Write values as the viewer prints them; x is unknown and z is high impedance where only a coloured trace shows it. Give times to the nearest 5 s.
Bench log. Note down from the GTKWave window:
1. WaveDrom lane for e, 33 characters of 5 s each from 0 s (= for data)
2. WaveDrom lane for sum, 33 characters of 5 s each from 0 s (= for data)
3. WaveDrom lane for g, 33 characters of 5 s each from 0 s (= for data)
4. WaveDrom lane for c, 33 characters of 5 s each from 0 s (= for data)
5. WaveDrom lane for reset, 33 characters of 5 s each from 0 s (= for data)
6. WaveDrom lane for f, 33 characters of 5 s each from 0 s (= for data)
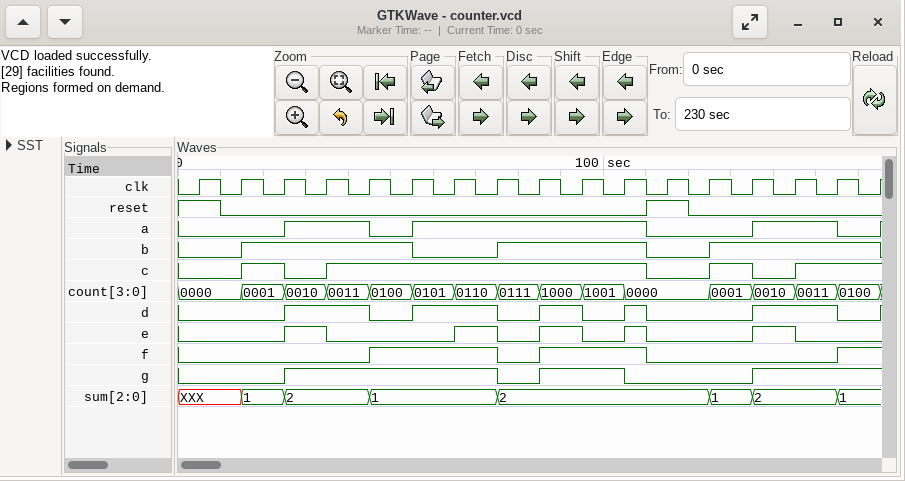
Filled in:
{name: 'e', wave: '0....1.0.....1.0.1.0.10....1.0...'}
{name: 'sum', wave: 'x..=.=...=.....=.........=.=...=.', data: '1 2 1 2 1 2 1'}
{name: 'g', wave: '0....1.........0.1...0.....1.....'}
{name: 'c', wave: '0..1.0.1..............0..1.0.1...'}
{name: 'reset', wave: '1.0...................1.0........'}
{name: 'f', wave: '0........1.....0.1....0........1.'}
